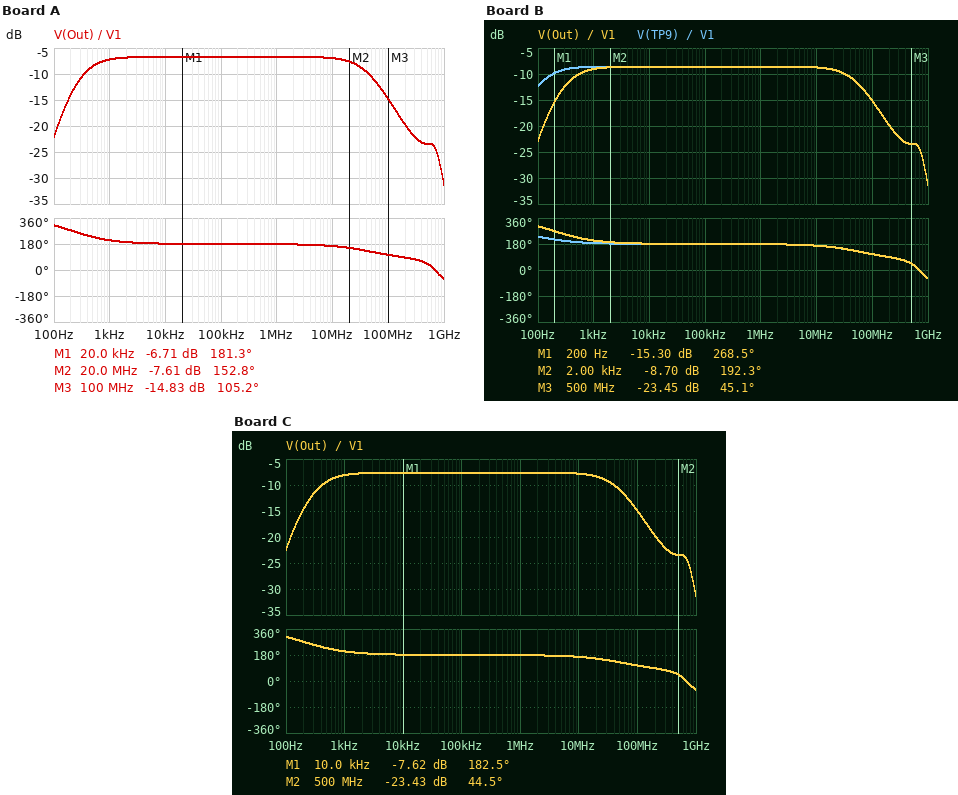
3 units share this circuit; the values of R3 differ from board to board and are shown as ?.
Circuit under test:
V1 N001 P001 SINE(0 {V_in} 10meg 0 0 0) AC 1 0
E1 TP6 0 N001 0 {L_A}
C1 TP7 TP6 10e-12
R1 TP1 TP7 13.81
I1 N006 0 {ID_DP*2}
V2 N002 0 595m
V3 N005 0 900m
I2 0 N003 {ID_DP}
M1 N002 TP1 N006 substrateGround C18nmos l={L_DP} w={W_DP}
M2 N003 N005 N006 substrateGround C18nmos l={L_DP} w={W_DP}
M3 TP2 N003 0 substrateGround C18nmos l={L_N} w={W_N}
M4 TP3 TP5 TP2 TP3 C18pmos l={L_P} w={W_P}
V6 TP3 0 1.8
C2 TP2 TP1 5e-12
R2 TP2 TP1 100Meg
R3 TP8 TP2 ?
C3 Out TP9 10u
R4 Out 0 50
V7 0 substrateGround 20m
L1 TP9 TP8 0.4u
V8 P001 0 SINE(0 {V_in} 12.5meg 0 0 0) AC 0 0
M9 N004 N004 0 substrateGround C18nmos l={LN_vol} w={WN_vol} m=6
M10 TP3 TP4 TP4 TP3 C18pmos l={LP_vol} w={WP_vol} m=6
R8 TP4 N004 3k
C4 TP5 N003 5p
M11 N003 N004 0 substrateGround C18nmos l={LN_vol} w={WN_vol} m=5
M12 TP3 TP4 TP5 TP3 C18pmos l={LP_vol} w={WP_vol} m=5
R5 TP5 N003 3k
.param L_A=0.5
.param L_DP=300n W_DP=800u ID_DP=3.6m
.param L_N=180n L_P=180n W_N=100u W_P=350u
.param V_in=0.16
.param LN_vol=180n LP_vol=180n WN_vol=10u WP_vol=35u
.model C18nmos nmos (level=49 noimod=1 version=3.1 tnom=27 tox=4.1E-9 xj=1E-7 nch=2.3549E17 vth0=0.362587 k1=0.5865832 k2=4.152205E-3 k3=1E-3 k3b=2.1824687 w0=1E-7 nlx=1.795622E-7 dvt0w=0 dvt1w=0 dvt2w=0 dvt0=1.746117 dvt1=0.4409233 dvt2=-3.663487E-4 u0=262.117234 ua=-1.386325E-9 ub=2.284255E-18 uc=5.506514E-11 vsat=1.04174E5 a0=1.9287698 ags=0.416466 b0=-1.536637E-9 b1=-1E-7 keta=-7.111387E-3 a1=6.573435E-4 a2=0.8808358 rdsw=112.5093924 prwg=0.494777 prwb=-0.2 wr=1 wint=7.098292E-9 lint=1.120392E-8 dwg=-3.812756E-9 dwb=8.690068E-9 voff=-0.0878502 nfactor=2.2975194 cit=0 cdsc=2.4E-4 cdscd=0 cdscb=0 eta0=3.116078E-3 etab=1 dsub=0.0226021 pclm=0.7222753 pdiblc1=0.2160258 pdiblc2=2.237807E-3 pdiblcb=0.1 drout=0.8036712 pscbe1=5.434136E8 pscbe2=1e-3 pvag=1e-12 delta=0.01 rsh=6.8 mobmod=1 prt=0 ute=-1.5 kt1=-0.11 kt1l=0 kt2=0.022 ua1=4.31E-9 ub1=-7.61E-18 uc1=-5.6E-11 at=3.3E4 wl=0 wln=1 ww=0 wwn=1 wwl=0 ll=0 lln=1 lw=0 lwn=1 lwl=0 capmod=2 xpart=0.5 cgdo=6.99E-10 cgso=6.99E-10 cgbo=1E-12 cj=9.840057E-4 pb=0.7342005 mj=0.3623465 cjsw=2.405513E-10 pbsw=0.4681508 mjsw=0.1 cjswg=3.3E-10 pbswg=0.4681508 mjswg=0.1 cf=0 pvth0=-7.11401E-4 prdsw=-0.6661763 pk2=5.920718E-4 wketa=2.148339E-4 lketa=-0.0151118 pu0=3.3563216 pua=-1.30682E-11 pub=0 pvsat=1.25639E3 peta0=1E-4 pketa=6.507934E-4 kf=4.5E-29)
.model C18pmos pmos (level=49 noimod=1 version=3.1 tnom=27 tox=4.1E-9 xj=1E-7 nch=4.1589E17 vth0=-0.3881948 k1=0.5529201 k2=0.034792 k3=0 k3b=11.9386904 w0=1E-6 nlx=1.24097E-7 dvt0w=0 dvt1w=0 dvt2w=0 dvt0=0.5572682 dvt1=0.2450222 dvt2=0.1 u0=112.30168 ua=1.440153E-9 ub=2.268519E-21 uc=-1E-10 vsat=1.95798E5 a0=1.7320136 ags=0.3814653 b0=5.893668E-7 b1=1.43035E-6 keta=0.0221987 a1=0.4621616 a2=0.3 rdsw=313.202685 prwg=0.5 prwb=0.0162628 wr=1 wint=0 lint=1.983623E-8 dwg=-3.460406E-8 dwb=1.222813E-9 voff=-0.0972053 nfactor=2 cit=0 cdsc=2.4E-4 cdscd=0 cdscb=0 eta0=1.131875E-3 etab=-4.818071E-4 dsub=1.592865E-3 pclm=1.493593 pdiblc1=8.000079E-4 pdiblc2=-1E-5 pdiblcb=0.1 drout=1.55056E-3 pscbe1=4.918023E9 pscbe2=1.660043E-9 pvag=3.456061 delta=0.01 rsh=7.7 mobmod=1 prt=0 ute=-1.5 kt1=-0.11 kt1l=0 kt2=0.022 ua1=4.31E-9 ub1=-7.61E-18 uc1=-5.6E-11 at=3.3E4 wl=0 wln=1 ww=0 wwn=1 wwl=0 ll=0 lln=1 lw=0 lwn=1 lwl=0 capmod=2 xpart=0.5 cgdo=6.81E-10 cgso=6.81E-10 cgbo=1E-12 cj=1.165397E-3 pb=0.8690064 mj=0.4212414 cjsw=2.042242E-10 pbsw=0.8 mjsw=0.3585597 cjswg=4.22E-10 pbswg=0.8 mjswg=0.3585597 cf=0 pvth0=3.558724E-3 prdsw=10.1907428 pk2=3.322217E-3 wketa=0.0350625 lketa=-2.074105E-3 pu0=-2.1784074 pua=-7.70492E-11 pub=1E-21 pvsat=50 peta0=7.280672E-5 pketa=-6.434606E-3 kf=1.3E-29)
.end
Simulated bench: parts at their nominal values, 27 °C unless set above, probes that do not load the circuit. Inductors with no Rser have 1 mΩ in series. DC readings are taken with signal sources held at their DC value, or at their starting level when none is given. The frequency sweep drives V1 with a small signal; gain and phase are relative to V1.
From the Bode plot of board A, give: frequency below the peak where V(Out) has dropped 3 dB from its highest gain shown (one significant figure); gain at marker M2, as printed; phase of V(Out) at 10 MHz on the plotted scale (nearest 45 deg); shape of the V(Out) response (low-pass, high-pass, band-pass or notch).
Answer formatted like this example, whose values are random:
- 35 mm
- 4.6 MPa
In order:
- 400 Hz
- -7.61 dB
- 180 deg
- band-pass
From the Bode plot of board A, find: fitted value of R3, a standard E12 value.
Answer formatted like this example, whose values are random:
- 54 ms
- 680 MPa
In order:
- 56 Ω
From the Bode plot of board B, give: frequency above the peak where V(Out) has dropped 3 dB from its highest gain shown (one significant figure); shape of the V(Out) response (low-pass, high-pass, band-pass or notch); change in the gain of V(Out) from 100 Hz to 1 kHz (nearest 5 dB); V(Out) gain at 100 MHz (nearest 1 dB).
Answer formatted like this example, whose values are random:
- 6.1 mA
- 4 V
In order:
- 50 MHz
- band-pass
- 15 dB
- -15 dB
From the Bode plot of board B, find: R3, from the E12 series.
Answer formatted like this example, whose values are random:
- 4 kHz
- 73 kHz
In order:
- 82 Ω
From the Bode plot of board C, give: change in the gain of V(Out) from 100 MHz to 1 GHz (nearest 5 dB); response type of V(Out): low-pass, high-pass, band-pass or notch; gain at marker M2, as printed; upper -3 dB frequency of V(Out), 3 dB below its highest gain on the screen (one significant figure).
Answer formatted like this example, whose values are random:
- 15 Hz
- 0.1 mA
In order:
- -15 dB
- band-pass
- -23.43 dB
- 50 MHz
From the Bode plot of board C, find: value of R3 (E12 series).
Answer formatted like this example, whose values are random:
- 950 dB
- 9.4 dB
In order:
- 68 Ω
